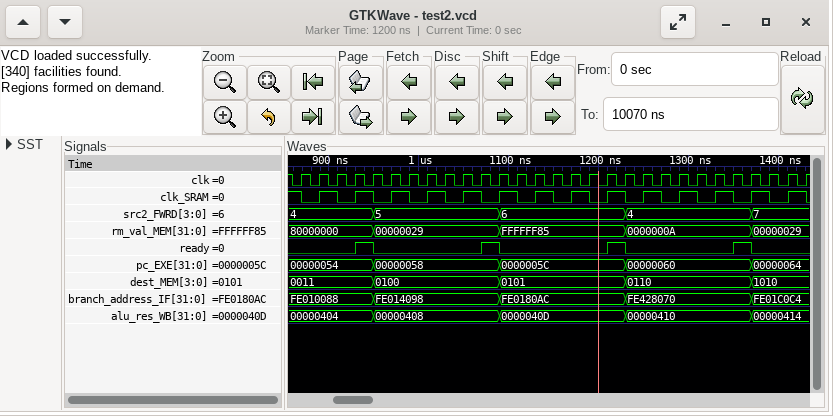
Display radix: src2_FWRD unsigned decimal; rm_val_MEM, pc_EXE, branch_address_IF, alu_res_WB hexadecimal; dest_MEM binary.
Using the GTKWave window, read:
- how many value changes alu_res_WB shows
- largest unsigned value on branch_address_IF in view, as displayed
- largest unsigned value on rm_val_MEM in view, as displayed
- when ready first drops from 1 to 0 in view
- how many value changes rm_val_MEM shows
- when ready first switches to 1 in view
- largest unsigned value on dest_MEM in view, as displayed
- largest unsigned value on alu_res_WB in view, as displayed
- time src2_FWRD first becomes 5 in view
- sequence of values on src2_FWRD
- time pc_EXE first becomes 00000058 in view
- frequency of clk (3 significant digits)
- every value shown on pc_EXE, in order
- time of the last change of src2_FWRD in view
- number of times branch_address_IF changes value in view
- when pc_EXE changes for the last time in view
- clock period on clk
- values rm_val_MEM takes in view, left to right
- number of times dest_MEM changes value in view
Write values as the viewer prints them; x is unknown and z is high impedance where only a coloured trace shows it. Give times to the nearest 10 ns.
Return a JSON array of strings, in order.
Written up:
["4", "FE428070", "FFFFFF85", "950 ns", "4", "930 ns", "1010", "00000414", "950 ns", "4, 5, 6, 4, 7", "950 ns", "50.0 MHz", "00000054, 00000058, 0000005C, 00000060, 00000064", "1370 ns", "4", "1370 ns", "20 ns", "80000000, 00000029, FFFFFF85, 0000000A, 00000029", "4"]
